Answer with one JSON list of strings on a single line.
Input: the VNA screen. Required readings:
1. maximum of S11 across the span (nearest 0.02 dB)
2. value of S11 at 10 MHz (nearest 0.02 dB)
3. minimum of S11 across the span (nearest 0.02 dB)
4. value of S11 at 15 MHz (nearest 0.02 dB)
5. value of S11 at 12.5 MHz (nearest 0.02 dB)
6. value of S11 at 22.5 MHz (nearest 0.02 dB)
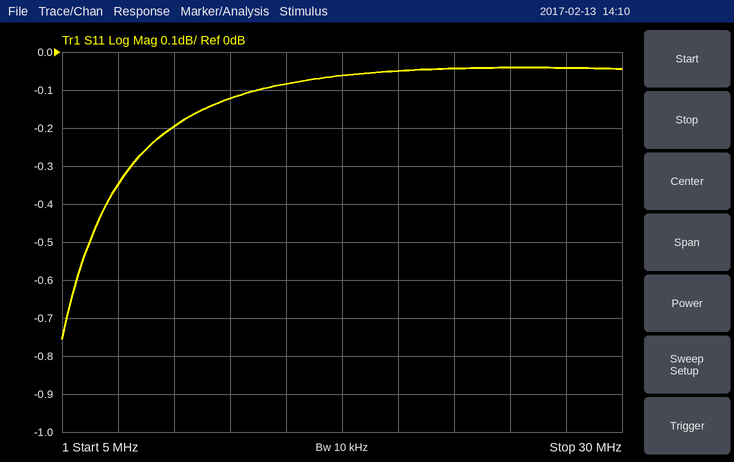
["-0.04 dB", "-0.20 dB", "-0.76 dB", "-0.08 dB", "-0.12 dB", "-0.04 dB"]
